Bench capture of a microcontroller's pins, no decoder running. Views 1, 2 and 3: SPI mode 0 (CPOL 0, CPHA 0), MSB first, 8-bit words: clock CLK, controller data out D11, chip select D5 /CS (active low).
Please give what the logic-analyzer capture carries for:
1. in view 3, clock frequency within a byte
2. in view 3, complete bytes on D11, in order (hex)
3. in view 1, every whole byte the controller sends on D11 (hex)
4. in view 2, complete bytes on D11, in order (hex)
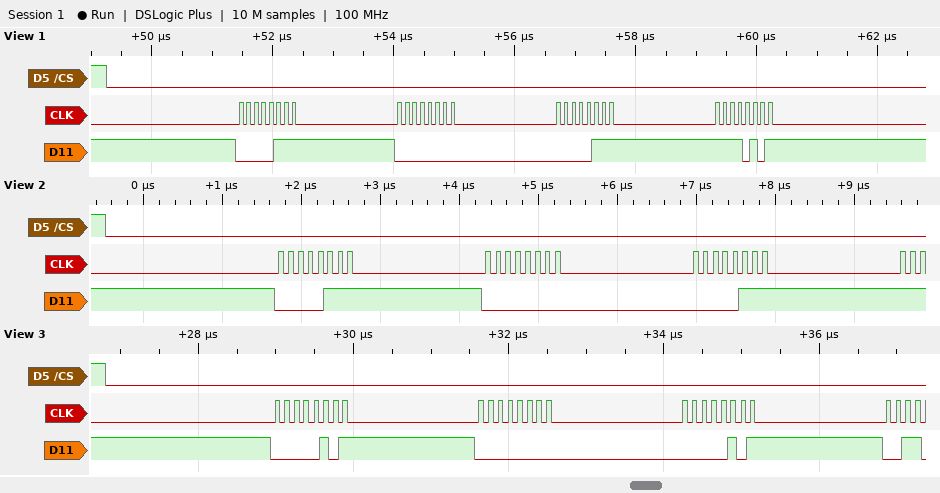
8 MHz
05 00 05
0x07 0x00 0x07 0xF5
07 00 07
